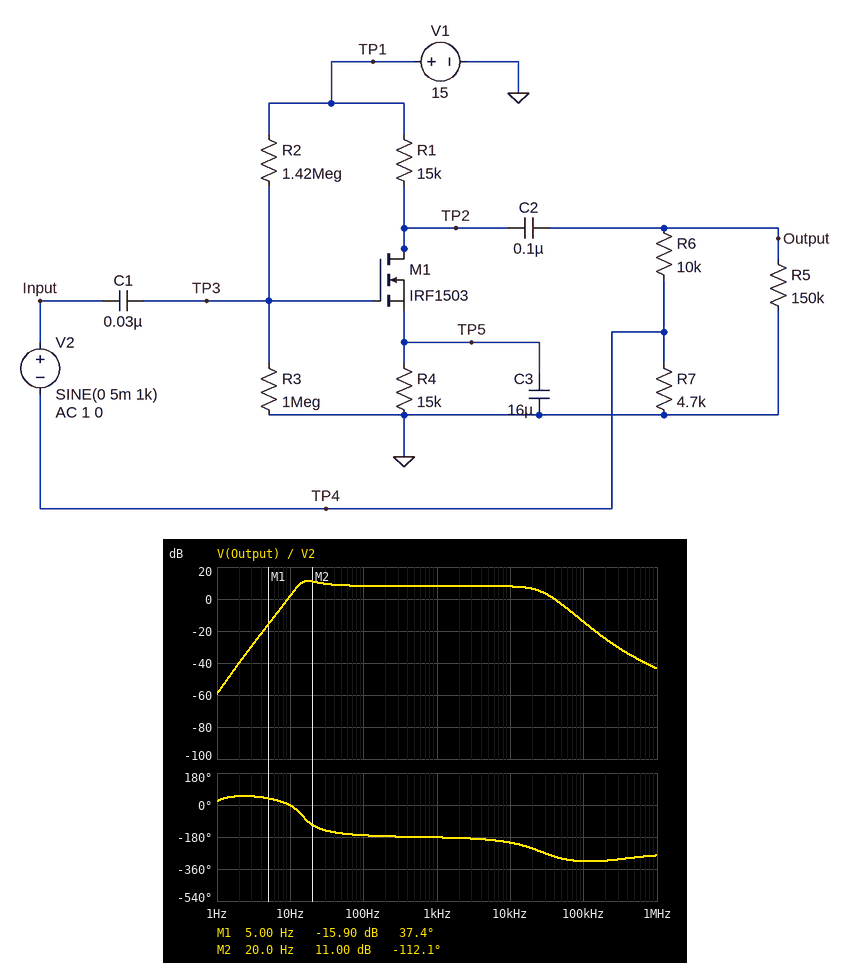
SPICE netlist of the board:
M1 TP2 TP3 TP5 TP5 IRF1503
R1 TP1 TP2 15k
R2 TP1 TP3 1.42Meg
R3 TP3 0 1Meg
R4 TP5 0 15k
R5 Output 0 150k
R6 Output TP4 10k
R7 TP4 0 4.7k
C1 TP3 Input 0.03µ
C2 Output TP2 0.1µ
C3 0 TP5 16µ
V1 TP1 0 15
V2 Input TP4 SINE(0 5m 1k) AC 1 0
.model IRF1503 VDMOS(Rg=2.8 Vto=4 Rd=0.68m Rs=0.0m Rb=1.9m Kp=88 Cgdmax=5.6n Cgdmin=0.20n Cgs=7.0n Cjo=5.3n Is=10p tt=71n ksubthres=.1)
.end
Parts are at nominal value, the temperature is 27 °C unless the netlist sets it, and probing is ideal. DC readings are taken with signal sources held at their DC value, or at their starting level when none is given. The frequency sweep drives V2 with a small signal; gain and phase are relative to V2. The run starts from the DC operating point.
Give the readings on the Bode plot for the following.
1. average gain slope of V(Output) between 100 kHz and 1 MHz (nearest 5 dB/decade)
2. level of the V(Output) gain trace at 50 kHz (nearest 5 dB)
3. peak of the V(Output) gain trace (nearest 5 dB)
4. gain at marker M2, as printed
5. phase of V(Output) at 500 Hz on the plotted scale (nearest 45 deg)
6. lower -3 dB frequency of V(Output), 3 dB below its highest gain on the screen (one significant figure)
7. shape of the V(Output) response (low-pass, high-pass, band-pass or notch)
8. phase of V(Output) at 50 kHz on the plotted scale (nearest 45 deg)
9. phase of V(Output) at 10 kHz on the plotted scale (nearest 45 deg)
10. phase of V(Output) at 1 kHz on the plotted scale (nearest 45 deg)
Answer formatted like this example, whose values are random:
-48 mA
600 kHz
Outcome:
-30 dB/decade
-5 dB
10 dB
11.00 dB
-180 deg
10 Hz
band-pass
-315 deg
-225 deg
-180 deg
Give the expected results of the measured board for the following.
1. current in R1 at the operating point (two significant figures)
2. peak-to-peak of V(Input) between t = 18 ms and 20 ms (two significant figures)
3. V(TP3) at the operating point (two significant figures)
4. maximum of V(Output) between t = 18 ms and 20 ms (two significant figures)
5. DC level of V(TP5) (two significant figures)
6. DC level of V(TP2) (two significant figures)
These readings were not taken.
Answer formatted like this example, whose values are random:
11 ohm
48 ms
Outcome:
170 µA
1.8 mV
6.2 V
13 mV
2.6 V
12 V
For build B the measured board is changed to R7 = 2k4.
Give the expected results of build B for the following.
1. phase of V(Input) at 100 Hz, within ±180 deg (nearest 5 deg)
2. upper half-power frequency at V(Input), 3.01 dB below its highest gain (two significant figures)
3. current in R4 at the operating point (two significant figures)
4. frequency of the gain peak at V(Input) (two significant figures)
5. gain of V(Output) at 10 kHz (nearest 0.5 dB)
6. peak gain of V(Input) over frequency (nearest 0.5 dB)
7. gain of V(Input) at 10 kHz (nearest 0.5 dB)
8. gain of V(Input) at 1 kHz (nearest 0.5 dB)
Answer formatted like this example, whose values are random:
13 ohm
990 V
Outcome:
-35 deg
29 Hz
170 µA
16 Hz
11.0 dB
2.5 dB
-10.5 dB
-11.0 dB
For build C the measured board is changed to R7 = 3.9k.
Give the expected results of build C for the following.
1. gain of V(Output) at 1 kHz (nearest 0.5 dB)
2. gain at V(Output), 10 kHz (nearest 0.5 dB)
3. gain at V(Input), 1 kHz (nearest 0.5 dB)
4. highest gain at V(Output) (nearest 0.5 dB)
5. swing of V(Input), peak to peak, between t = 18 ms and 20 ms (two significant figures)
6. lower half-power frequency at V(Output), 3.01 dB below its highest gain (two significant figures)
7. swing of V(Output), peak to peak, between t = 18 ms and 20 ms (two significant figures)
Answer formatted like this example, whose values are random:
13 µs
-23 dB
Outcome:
9.0 dB
8.5 dB
-14.0 dB
11.0 dB
2.0 mV
14 Hz
28 mV
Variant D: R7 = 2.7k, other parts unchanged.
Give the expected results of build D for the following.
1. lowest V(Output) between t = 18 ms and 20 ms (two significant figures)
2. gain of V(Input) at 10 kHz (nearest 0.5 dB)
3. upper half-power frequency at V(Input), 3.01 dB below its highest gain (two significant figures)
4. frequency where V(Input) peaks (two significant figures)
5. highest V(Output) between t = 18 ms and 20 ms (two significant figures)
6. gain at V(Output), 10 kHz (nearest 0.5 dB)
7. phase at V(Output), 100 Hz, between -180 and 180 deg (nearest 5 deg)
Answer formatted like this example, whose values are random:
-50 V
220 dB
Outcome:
-17 mV
-11.0 dB
27 Hz
16 Hz
17 mV
10.5 dB
-165 deg
